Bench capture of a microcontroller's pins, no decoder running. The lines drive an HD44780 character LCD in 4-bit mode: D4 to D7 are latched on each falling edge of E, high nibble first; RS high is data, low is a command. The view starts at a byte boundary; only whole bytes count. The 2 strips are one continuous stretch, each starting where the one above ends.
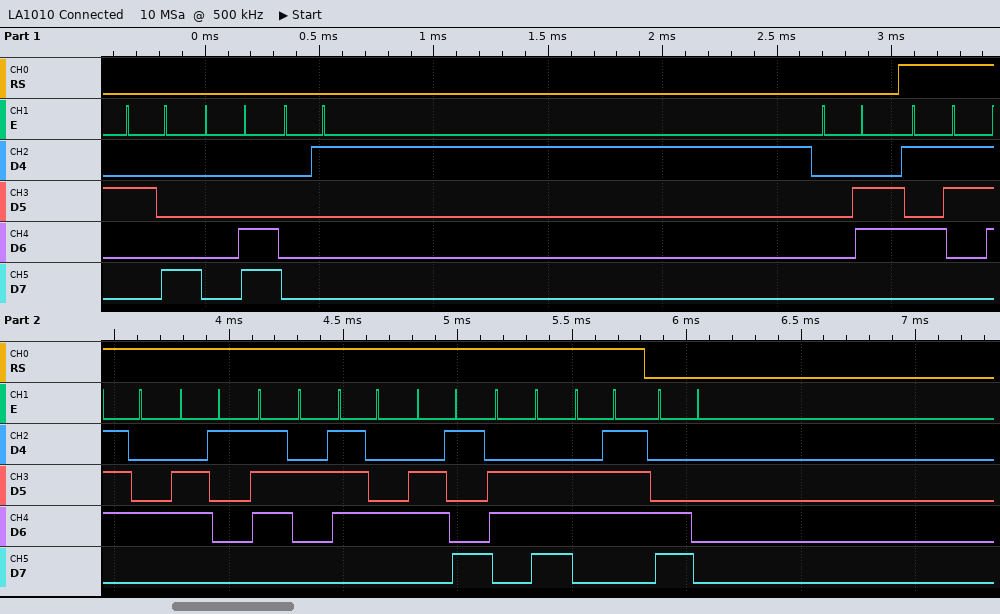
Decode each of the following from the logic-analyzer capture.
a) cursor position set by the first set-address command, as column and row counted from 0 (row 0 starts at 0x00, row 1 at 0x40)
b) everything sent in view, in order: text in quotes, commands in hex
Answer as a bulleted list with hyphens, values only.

- column 0, row 1
- 0x28 0x0C 0x01 0x06 "Starting" 0xC0
